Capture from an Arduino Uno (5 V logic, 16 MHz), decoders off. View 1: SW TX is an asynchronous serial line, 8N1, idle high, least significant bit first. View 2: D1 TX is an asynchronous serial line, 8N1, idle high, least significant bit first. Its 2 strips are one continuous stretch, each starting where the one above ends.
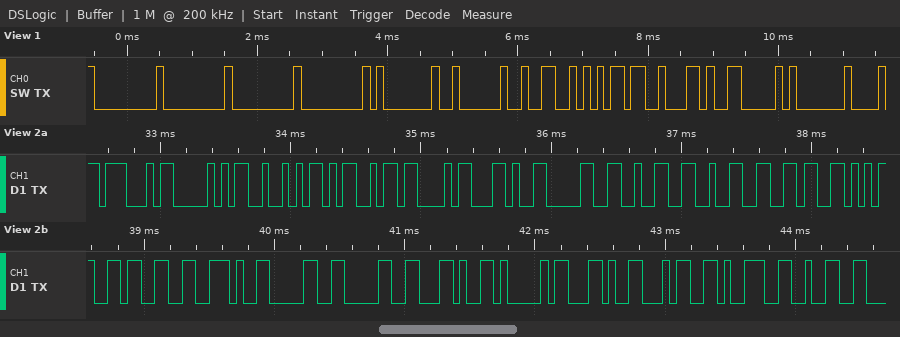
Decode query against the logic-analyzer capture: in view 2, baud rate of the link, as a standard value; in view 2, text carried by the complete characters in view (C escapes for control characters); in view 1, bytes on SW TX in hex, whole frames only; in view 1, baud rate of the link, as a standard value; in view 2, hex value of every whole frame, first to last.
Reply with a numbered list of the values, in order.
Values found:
1. 19200 baud
2. "GPRMC,022653.00,A,492"
3. 00 00 00 00 01 02 32 B5 62 06 01
4. 9600 baud
5. 0x47 0x50 0x52 0x4D 0x43 0x2C 0x30 0x32 0x32 0x36 0x35 0x33 0x2E 0x30 0x30 0x2C 0x41 0x2C 0x34 0x39 0x32
